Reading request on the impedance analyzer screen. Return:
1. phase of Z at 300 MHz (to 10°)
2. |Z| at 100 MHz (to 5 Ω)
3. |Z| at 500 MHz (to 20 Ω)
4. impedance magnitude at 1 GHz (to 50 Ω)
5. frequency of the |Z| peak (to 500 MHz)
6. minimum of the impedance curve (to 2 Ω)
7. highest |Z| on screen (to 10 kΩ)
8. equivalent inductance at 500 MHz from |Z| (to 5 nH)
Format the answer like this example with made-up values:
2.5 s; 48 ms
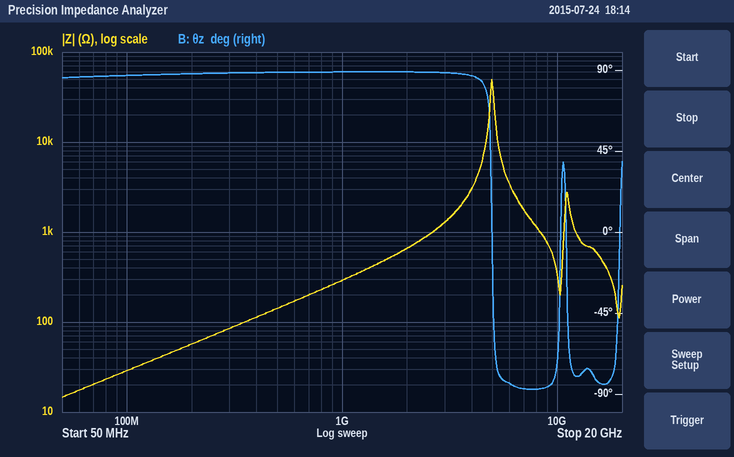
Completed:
90°; 30 Ω; 140 Ω; 300 Ω; 5.0 GHz; 14 Ω; 50 kΩ; 45 nH
